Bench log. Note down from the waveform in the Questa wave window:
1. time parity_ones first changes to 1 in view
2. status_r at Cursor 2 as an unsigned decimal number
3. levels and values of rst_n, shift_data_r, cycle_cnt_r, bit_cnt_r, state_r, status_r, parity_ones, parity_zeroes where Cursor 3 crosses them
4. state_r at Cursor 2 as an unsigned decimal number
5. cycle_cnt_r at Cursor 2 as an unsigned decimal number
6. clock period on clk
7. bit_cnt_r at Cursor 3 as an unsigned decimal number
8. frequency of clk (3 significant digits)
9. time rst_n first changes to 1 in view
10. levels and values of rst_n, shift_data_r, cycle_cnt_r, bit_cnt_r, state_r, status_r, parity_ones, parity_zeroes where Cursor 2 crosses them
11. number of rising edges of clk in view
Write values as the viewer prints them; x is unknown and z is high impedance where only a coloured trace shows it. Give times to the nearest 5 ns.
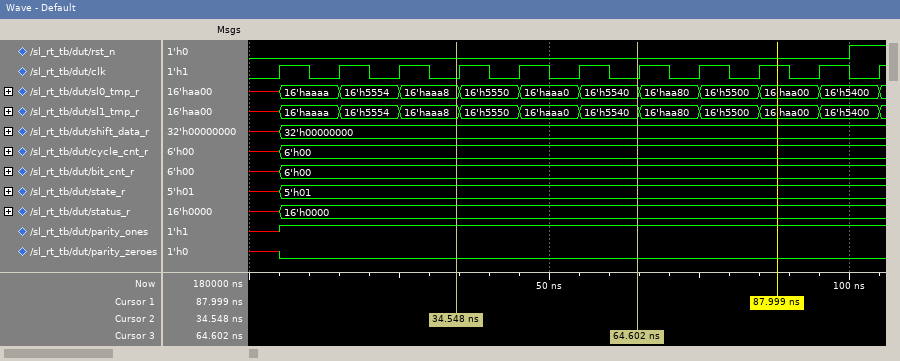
5 ns
0
rst_n=0, shift_data_r=32'h00000000, cycle_cnt_r=6'h00, bit_cnt_r=6'h00, state_r=5'h01, status_r=16'h0000, parity_ones=1, parity_zeroes=0
1
0
10 ns
0
100 MHz
100 ns
rst_n=0, shift_data_r=32'h00000000, cycle_cnt_r=6'h00, bit_cnt_r=6'h00, state_r=5'h01, status_r=16'h0000, parity_ones=1, parity_zeroes=0
11
